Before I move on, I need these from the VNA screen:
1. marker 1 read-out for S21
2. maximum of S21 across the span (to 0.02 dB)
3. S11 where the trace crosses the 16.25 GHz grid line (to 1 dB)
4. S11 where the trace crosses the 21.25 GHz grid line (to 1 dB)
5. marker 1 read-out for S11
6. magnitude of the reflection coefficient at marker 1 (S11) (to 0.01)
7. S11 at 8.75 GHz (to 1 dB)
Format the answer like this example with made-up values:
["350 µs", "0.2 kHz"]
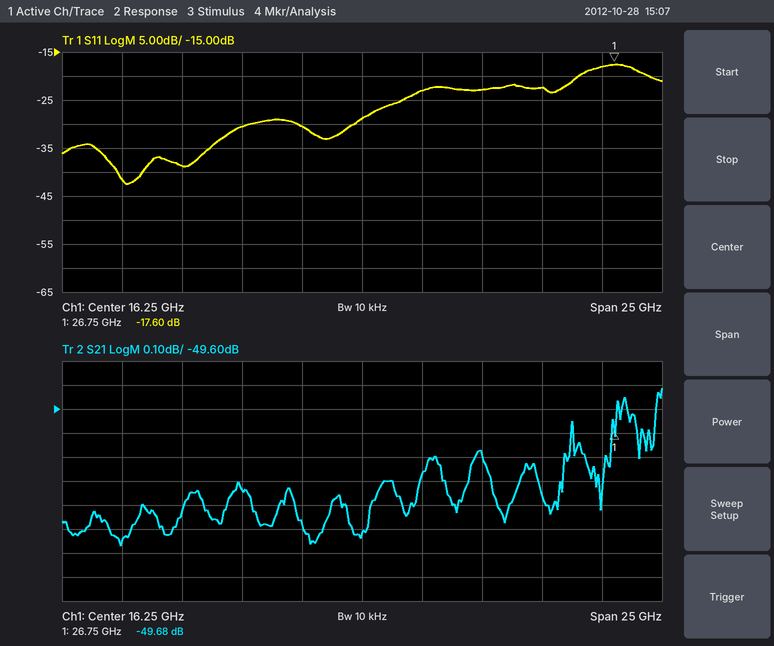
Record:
["-49.68 dB", "-49.52 dB", "-29 dB", "-23 dB", "-17.60 dB", "0.13", "-39 dB"]
